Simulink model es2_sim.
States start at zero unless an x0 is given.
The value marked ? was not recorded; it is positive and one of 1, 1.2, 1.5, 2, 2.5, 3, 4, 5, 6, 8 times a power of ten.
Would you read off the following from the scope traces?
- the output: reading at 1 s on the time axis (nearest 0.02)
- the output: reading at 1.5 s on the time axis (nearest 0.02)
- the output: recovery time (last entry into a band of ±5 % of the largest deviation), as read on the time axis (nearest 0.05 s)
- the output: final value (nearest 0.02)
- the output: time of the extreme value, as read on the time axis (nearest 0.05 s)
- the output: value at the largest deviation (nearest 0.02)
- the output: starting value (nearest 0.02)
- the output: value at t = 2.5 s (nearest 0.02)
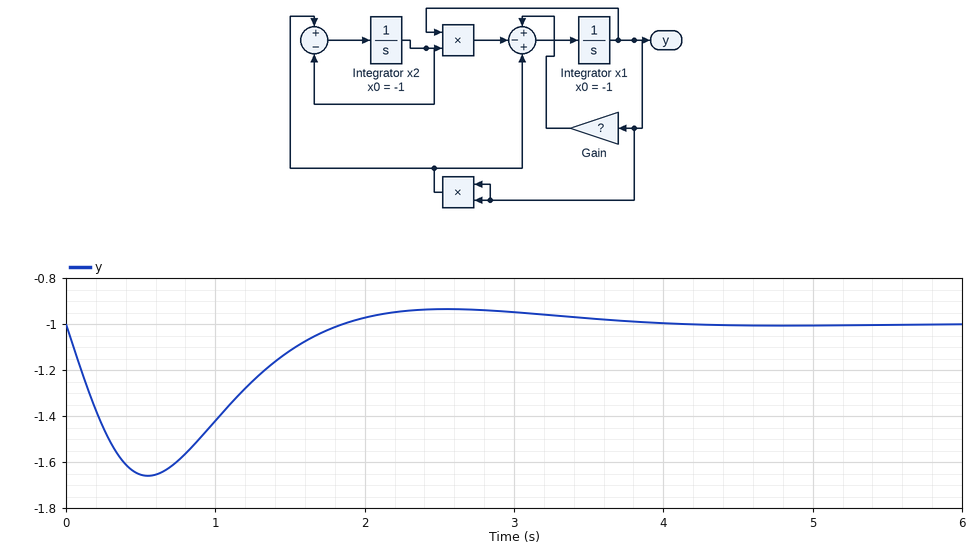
-1.42
-1.12
3.35 s
-1.00
0.55 s
-1.66
-1.00
-0.94
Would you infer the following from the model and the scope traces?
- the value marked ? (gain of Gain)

2
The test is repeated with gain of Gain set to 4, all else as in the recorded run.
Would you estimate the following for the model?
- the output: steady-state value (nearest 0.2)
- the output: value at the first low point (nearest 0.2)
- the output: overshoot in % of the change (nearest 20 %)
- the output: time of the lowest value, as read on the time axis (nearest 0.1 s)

-1.6
-2.8
200 %
0.5 s
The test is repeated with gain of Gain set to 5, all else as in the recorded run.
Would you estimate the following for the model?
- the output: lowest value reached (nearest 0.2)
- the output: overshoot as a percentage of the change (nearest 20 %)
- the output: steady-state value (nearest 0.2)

-3.2
180 %
-1.8
